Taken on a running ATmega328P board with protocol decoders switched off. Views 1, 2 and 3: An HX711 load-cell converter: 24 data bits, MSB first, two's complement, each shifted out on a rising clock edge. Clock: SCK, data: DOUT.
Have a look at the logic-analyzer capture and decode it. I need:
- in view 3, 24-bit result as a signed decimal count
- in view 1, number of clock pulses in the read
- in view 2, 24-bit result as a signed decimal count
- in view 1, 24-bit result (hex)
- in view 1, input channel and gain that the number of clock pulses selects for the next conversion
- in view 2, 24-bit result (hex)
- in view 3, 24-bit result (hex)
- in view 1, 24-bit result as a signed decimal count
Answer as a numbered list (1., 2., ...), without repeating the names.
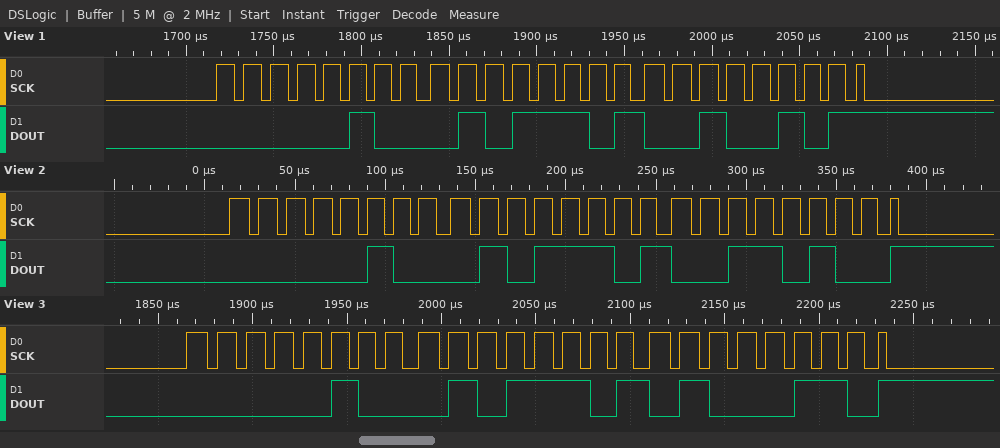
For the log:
1. 286022
2. 25
3. 286004
4. 0x045D25
5. channel A, gain 128
6. 0x045D34
7. 0x045D46
8. 285989
